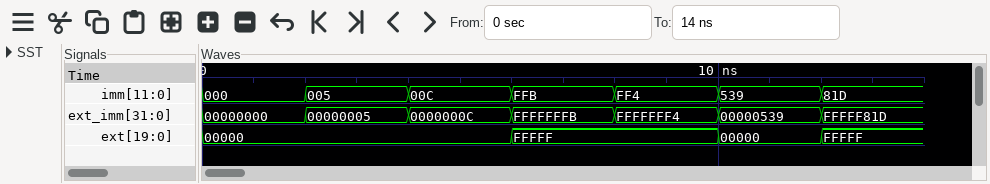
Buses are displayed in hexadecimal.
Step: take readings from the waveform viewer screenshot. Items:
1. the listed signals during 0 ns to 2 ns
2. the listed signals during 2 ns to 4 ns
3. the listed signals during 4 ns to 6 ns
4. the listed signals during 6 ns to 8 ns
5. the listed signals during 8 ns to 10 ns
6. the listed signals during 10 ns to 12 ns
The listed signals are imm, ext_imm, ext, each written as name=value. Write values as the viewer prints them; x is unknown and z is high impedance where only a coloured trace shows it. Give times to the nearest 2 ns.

imm=000, ext_imm=00000000, ext=00000
imm=005, ext_imm=00000005, ext=00000
imm=00C, ext_imm=0000000C, ext=00000
imm=FFB, ext_imm=FFFFFFFB, ext=FFFFF
imm=FF4, ext_imm=FFFFFFF4, ext=FFFFF
imm=539, ext_imm=00000539, ext=00000
